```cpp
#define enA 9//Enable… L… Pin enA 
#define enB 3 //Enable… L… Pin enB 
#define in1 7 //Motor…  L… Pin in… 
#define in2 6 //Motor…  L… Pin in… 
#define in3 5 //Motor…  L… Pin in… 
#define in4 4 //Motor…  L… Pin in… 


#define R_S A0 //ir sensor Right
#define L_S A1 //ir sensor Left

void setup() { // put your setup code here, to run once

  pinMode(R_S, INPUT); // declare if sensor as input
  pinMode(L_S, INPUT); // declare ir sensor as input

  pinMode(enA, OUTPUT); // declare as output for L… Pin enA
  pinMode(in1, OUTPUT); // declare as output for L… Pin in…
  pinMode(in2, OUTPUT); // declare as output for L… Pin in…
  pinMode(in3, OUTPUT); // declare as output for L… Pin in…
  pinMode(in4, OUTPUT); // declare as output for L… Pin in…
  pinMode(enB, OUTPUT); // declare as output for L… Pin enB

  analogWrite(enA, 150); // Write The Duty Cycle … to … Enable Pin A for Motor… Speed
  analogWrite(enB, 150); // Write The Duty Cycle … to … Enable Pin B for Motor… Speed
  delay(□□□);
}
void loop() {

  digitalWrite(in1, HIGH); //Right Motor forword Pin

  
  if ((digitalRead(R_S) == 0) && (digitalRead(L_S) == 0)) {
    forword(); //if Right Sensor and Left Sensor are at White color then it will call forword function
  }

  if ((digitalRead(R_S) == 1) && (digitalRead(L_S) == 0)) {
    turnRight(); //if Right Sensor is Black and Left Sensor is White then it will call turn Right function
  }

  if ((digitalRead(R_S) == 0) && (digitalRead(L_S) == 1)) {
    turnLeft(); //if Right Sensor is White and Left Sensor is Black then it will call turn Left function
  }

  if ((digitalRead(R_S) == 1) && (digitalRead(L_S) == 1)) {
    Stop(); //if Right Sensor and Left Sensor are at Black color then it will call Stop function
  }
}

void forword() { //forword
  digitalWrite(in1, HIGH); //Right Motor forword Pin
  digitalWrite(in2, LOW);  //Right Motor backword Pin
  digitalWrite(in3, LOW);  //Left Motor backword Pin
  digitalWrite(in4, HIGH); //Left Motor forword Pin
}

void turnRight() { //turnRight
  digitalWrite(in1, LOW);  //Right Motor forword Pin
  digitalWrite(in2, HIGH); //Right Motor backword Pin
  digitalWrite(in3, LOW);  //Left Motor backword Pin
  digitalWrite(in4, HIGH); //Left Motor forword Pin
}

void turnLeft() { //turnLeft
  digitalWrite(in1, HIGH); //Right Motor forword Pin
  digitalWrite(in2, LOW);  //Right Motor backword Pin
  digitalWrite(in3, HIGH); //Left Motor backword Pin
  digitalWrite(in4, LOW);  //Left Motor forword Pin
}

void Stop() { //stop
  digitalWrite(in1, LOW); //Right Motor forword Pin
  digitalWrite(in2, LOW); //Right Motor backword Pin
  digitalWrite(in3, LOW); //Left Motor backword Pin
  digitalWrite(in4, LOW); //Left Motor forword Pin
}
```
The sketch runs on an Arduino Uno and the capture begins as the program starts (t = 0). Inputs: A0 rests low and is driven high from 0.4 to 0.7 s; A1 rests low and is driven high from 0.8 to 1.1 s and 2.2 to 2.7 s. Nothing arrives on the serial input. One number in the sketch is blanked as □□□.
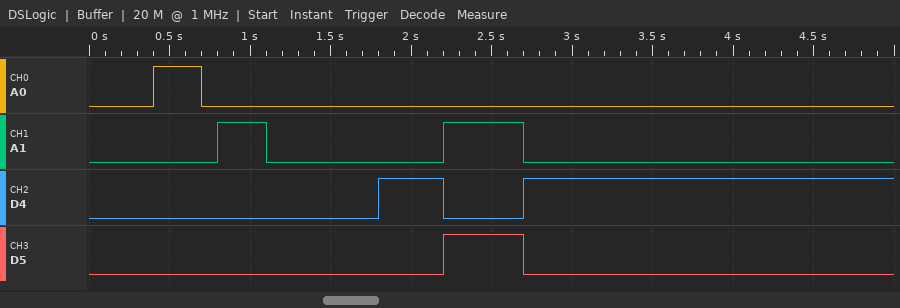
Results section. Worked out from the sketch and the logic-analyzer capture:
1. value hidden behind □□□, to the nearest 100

1800
